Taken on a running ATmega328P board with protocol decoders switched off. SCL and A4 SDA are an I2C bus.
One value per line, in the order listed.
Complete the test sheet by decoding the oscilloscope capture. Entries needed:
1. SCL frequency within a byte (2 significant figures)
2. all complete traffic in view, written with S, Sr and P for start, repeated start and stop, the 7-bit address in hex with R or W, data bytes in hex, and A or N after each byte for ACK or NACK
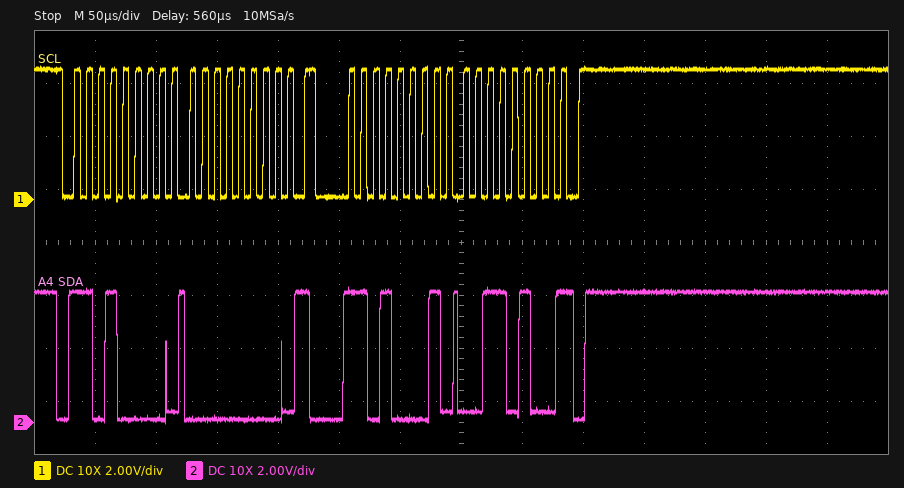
100 kHz
S 68W A 00 A Sr 68R A 34 N P
